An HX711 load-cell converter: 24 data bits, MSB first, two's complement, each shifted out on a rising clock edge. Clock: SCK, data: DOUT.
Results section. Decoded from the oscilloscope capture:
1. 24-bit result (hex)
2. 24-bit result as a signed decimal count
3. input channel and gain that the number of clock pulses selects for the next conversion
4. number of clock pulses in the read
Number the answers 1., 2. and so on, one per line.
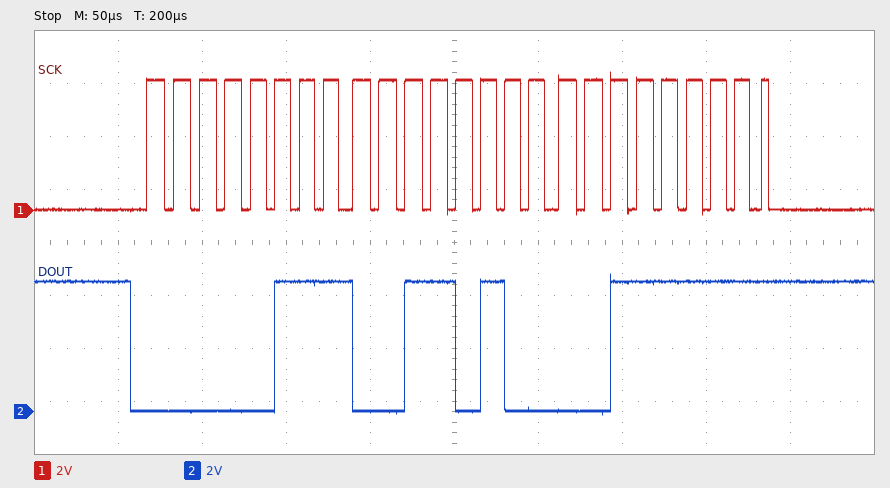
1. 0x07343F
2. 472127
3. channel A, gain 128
4. 25
